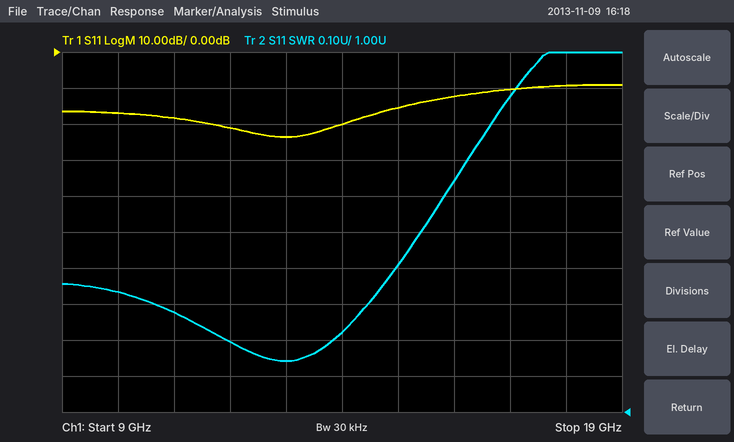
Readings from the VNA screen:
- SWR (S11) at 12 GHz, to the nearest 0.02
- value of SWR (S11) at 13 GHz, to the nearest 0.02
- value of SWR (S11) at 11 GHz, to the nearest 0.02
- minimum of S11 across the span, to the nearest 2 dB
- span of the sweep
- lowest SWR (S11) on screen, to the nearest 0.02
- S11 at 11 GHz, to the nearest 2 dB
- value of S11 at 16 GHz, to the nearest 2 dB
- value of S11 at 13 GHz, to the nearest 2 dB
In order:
1.20
1.14
1.28
-24 dB
10 GHz
1.14
-18 dB
-12 dB
-24 dB
